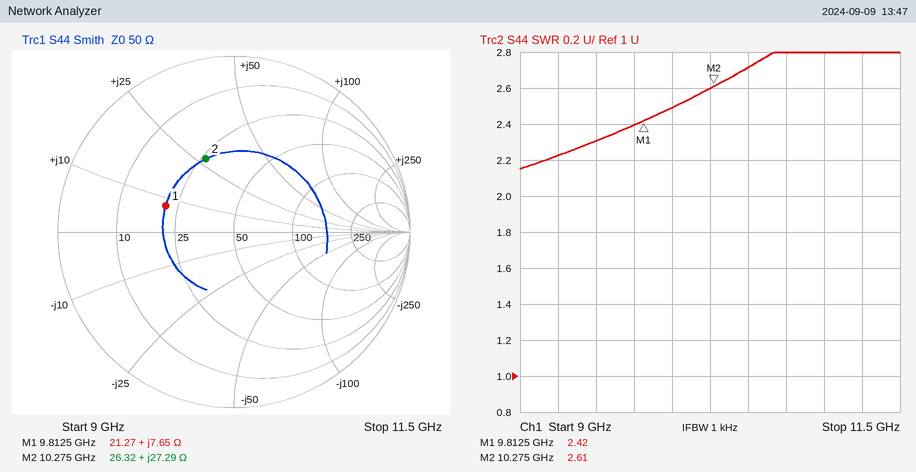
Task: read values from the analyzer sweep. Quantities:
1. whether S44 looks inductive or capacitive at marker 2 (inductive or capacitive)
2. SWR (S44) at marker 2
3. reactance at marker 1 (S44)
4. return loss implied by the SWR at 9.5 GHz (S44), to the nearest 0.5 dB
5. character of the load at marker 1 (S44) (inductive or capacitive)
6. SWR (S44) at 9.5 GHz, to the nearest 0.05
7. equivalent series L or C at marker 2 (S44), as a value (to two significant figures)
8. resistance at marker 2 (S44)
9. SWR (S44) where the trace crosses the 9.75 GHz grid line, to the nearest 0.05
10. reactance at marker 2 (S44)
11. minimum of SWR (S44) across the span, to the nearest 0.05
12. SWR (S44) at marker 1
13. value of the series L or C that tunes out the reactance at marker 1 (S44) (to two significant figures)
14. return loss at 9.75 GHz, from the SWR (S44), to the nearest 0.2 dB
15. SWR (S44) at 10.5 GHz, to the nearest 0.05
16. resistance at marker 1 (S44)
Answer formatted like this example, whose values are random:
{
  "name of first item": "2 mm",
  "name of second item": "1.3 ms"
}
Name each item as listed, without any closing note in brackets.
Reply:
{
  "whether S44 looks inductive or capacitive at marker 2": "inductive",
  "SWR (S44) at marker 2": "2.61",
  "reactance at marker 1": "+7.65 Ω",
  "return loss implied by the SWR at 9.5 GHz (S44), to the nearest 0.5 dB": "8.0 dB",
  "character of the load at marker 1 (S44)": "inductive",
  "SWR (S44) at 9.5 GHz, to the nearest 0.05": "2.30",
  "equivalent series L or C at marker 2 (S44), as a value": "420 pH",
  "resistance at marker 2": "26.32 Ω",
  "SWR (S44) where the trace crosses the 9.75 GHz grid line, to the nearest 0.05": "2.40",
  "reactance at marker 2": "+27.29 Ω",
  "minimum of SWR (S44) across the span, to the nearest 0.05": "2.15",
  "SWR (S44) at marker 1": "2.42",
  "value of the series L or C that tunes out the reactance at marker 1 (S44)": "2.1 pF",
  "return loss at 9.75 GHz, from the SWR (S44), to the nearest 0.2 dB": "7.8 dB",
  "SWR (S44) at 10.5 GHz, to the nearest 0.05": "2.70",
  "resistance at marker 1": "21.27 Ω"
}
